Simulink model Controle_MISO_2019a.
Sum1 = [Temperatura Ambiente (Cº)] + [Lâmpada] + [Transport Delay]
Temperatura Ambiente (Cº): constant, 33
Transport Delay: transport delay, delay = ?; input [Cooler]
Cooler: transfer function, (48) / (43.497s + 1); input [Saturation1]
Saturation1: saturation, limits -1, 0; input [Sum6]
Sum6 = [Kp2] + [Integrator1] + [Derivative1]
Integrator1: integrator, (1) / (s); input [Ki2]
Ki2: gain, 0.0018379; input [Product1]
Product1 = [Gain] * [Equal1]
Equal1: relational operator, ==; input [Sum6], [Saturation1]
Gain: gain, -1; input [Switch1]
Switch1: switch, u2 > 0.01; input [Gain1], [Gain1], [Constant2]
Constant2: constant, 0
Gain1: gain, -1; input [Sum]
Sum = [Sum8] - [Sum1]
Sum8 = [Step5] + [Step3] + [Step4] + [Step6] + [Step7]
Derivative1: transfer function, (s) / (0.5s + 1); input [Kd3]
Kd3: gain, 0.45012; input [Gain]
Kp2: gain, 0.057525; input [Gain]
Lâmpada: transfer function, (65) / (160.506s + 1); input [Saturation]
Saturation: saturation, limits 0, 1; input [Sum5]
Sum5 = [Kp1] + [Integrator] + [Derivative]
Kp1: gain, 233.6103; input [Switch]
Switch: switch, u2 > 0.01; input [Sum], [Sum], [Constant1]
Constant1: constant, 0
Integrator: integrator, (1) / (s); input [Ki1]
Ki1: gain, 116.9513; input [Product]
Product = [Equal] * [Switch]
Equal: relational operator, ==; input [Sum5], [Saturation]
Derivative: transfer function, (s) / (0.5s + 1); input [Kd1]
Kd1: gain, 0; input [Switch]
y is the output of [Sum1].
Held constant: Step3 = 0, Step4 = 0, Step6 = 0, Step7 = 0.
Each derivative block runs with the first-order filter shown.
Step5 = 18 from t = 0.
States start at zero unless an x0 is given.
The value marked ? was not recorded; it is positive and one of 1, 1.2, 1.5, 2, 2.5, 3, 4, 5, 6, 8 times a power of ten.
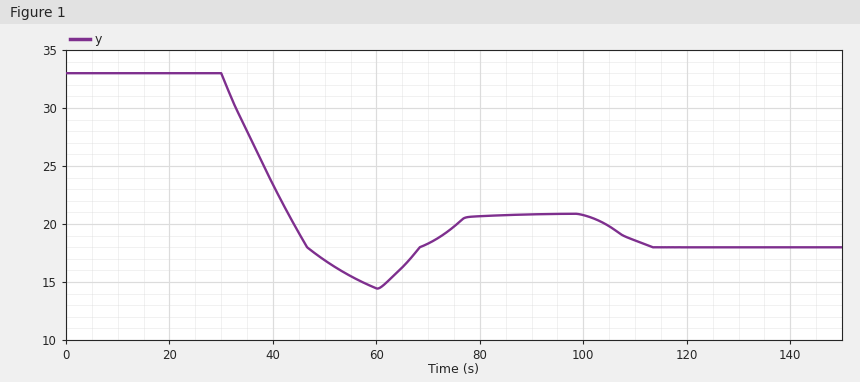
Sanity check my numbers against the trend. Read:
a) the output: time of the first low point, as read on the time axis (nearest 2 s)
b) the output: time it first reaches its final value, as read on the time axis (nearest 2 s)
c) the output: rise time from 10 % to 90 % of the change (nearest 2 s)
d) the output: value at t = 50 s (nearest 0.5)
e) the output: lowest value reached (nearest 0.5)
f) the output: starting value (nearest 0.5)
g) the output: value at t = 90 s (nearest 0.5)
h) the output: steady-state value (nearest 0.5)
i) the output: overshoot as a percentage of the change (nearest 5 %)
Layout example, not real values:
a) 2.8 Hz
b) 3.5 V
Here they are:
a) 60 s
b) 46 s
c) 14 s
d) 17.0
e) 14.5
f) 33.0
g) 21.0
h) 18.0
i) 25 %
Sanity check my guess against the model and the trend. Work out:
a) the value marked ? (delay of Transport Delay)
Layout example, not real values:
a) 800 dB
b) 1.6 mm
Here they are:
a) 30
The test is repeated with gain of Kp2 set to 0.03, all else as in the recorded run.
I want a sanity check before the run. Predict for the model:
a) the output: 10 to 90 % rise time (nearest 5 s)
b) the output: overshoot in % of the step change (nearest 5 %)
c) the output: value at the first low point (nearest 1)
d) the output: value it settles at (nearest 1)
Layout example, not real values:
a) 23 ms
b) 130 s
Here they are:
a) 20 s
b) 15 %
c) 16
d) 18
